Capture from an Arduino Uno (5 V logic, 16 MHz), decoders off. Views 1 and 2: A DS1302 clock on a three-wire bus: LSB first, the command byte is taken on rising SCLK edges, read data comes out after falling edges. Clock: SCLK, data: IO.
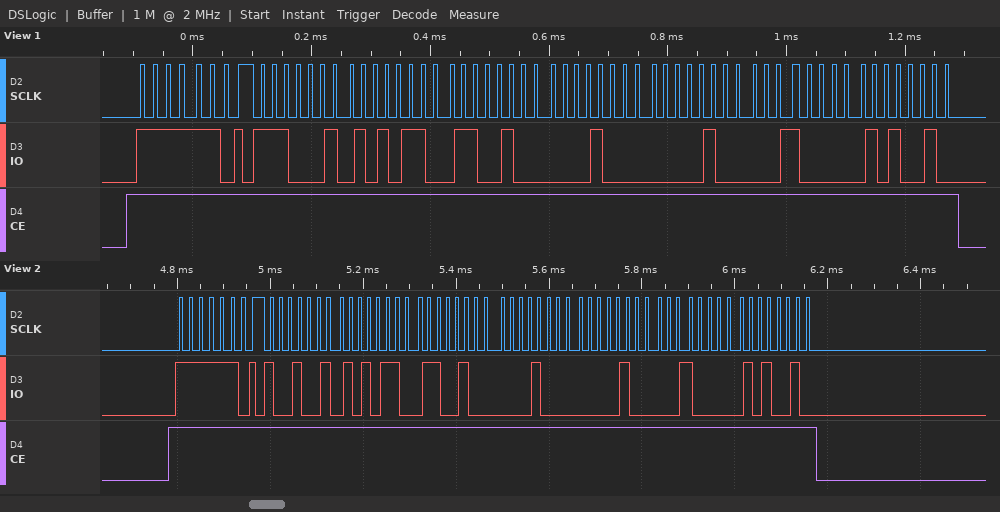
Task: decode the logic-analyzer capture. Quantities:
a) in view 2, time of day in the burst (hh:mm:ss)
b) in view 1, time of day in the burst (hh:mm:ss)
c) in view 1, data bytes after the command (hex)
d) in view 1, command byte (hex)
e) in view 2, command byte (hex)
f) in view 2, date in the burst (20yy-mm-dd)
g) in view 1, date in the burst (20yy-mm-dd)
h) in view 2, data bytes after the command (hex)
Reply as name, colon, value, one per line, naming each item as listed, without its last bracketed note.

in view 2, time of day in the burst: 13:35:49
in view 1, time of day in the burst: 13:35:47
in view 1, data bytes after the command: 47 35 13 08 10 04 25
in view 1, command byte: 0xBF
in view 2, command byte: 0xBF
in view 2, date in the burst: 2025-10-08
in view 1, date in the burst: 2025-10-08
in view 2, data bytes after the command: 49 35 13 08 10 04 25
